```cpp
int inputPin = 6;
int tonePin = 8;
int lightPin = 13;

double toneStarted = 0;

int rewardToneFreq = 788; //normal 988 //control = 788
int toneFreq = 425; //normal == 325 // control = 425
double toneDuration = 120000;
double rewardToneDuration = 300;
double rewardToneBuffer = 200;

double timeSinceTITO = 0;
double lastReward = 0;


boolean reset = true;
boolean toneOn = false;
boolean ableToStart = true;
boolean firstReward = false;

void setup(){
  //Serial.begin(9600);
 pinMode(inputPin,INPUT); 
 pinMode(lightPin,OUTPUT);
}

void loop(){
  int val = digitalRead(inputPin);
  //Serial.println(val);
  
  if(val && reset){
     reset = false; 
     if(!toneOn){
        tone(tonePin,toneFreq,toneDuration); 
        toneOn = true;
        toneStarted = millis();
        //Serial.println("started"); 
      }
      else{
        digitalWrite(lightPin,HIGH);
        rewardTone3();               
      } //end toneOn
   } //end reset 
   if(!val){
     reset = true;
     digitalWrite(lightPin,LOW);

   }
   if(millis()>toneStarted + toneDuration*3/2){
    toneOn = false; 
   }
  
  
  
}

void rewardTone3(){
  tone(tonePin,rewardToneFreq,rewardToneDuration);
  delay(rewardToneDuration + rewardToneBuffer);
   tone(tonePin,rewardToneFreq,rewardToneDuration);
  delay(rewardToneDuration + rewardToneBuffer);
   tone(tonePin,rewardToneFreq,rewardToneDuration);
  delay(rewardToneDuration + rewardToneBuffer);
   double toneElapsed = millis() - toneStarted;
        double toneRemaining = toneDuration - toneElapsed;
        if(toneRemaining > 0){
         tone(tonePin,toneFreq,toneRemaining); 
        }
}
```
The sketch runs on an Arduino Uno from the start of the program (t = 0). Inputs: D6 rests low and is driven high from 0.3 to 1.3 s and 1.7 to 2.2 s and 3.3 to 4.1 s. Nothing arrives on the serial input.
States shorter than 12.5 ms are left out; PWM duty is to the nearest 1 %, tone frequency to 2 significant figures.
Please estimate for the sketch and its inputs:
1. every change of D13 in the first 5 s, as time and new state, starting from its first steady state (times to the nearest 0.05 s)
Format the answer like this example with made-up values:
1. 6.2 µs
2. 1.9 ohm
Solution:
1. 0 s low; 1.7 s high; 3.2 s low; 3.3 s high; 4.8 s low
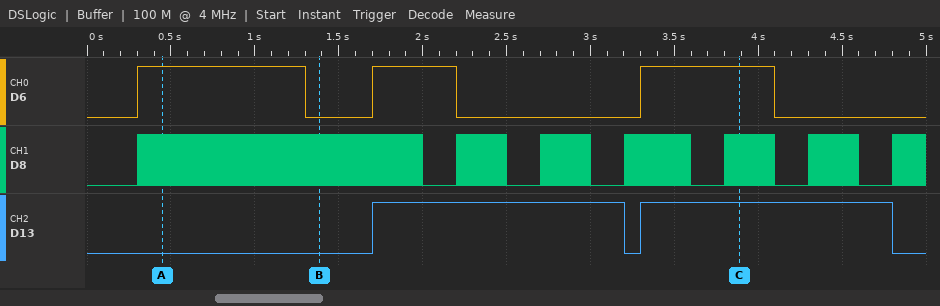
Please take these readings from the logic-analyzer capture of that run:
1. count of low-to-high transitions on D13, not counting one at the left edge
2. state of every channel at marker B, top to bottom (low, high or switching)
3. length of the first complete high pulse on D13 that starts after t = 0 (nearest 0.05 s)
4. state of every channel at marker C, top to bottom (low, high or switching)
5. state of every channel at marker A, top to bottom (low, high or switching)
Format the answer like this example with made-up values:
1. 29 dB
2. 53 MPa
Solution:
1. 2
2. D6 low, D8 switching, D13 low
3. 1.50 s
4. D6 high, D8 switching, D13 high
5. D6 high, D8 switching, D13 low
